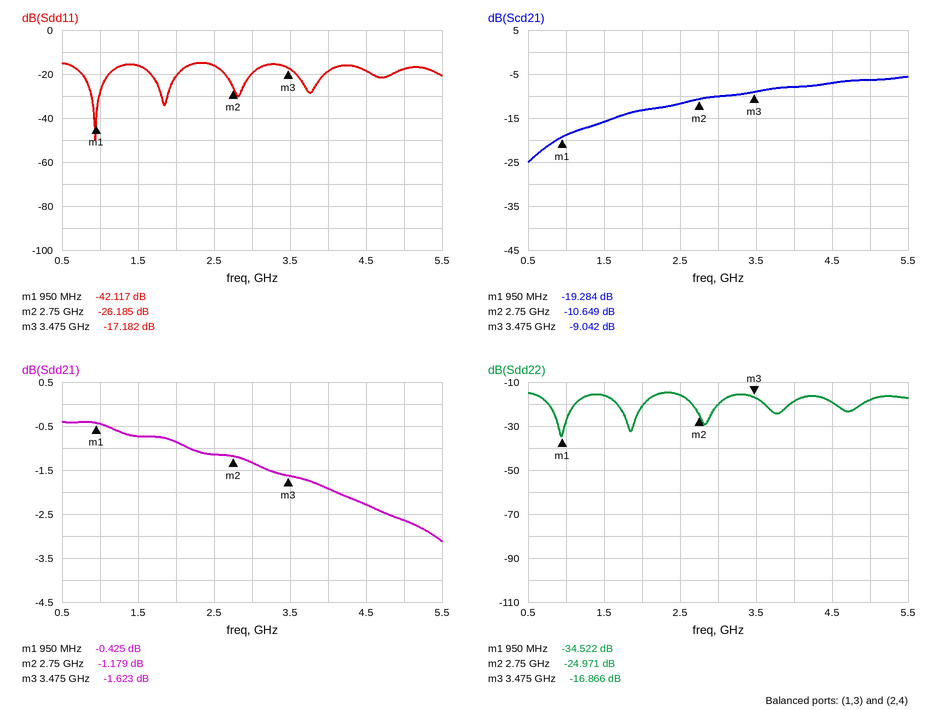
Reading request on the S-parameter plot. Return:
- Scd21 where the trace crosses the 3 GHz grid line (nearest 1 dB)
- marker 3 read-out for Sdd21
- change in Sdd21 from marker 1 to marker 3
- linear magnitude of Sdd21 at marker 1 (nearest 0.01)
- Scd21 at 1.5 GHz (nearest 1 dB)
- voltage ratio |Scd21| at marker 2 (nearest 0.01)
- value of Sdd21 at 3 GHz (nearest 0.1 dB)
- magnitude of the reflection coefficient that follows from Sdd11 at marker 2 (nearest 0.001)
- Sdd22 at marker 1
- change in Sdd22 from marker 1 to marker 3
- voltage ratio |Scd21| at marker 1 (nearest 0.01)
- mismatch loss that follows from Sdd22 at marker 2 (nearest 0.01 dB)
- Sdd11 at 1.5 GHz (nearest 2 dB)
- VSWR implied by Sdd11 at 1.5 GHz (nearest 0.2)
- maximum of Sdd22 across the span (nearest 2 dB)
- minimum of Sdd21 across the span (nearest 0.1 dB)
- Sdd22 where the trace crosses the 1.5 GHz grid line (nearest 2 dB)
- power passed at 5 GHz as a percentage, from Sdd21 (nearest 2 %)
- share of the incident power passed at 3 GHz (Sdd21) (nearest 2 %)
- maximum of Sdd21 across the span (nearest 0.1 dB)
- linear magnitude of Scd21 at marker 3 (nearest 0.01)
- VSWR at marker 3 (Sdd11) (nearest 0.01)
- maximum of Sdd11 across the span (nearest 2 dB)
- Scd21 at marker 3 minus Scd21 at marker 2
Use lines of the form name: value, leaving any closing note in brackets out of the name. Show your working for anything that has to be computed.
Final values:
Scd21 where the trace crosses the 3 GHz grid line: -10 dB
marker 3 read-out for Sdd21: -1.623 dB
change in Sdd21 from marker 1 to marker 3: -1.623 − (-0.425) = -1.198 dB
linear magnitude of Sdd21 at marker 1: 10^(-0.425/20) ≈ 0.95
Scd21 at 1.5 GHz: -16 dB
voltage ratio |Scd21| at marker 2: 10^(-10.649/20) ≈ 0.29
value of Sdd21 at 3 GHz: -1.3 dB
magnitude of the reflection coefficient that follows from Sdd11 at marker 2: 10^(-26.185/20) ≈ 0.049
Sdd22 at marker 1: -34.522 dB
change in Sdd22 from marker 1 to marker 3: -16.866 − (-34.522) = 17.656 dB
voltage ratio |Scd21| at marker 1: 10^(-19.284/20) ≈ 0.11
mismatch loss that follows from Sdd22 at marker 2: −10 log10(1 − 10^(-24.971/10)) ≈ 0.01 dB
Sdd11 at 1.5 GHz: -16 dB
VSWR implied by Sdd11 at 1.5 GHz: |Γ| = 10^(-16/20) = 0.1585; VSWR = (1 + 0.1585)/(1 − 0.1585) ≈ 1.4
maximum of Sdd22 across the span: -14 dB
minimum of Sdd21 across the span: -3.1 dB
Sdd22 where the trace crosses the 1.5 GHz grid line: -16 dB
power passed at 5 GHz as a percentage, from Sdd21: 10^(-2.6/10) ≈ 55.0 %, so 54 % to the nearest 2 %
share of the incident power passed at 3 GHz (Sdd21): 10^(-1.3/10) ≈ 74 %
maximum of Sdd21 across the span: -0.4 dB
linear magnitude of Scd21 at marker 3: 10^(-9.042/20) ≈ 0.35
VSWR at marker 3 (Sdd11): (1 + 0.1383)/(1 − 0.1383) ≈ 1.32
maximum of Sdd11 across the span: -14 dB
Scd21 at marker 3 minus Scd21 at marker 2: -9.042 − (-10.649) = 1.607 dB
